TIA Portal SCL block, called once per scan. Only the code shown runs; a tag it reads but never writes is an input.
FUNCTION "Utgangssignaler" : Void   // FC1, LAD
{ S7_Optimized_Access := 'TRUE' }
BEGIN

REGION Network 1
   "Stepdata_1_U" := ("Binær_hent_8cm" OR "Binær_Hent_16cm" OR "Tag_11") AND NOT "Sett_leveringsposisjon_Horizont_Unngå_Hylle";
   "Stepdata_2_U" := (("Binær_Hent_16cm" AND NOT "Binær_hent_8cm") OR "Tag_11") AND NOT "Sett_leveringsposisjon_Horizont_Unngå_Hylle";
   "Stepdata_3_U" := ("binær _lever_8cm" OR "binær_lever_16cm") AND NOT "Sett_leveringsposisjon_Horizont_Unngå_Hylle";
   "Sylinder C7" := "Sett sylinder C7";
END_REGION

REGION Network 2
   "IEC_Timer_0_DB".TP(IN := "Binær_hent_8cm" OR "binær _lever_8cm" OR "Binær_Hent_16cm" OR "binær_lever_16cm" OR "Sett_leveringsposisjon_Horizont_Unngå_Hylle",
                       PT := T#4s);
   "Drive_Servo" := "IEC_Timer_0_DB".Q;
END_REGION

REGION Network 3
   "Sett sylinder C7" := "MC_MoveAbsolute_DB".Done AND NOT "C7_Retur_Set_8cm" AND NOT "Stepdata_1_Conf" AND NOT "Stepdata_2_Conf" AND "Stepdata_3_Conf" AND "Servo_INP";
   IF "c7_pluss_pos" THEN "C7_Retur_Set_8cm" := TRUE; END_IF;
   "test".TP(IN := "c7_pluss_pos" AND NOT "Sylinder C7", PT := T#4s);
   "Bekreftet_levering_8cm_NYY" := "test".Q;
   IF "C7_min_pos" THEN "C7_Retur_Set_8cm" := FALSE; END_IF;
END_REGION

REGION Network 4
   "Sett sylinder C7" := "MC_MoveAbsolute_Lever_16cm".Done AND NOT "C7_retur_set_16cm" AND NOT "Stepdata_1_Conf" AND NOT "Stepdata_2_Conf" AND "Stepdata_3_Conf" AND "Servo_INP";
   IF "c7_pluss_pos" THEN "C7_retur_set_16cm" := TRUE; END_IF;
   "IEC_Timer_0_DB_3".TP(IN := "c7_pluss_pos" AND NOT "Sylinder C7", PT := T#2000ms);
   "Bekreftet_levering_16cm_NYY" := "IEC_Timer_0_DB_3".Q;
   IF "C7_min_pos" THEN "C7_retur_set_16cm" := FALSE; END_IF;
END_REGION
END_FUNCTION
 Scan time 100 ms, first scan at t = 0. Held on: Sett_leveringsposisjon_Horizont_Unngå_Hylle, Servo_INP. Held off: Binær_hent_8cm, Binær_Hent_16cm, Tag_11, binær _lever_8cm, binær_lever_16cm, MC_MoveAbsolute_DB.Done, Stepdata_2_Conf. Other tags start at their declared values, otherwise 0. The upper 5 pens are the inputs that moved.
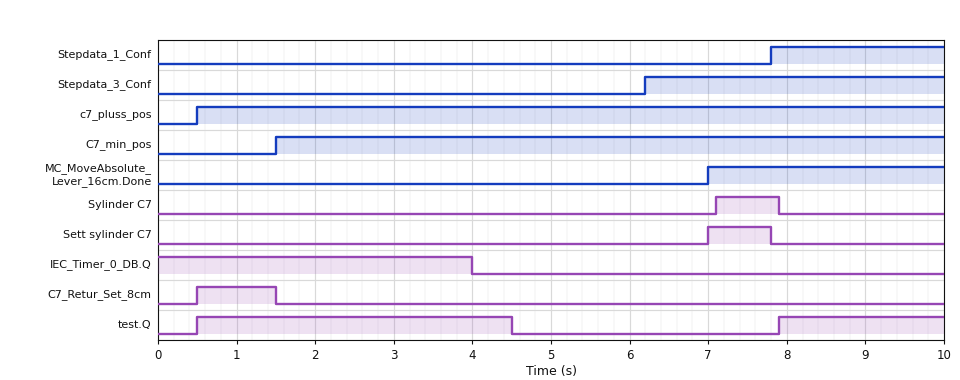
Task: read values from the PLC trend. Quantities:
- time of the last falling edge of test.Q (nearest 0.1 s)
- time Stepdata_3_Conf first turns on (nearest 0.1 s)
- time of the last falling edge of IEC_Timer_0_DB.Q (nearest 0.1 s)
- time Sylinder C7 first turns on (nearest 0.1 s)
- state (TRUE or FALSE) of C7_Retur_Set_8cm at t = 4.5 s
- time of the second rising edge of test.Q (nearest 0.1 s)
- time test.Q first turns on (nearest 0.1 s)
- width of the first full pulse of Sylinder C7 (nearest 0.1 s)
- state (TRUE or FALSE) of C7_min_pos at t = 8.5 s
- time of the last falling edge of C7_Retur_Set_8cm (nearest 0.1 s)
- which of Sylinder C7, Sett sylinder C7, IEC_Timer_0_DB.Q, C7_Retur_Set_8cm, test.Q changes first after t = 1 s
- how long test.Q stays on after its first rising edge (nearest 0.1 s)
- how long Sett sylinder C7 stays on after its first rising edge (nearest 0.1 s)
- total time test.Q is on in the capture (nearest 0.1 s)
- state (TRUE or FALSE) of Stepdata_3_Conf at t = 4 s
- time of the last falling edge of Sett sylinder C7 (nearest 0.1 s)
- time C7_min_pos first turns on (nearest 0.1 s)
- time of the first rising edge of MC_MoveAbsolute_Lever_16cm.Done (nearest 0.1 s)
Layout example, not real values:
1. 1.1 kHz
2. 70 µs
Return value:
1. 4.5 s
2. 6.2 s
3. 4.0 s
4. 7.1 s
5. FALSE
6. 7.9 s
7. 0.5 s
8. 0.8 s
9. TRUE
10. 1.5 s
11. C7_Retur_Set_8cm
12. 4.0 s
13. 0.8 s
14. 6.1 s
15. FALSE
16. 7.8 s
17. 1.5 s
18. 7.0 s
